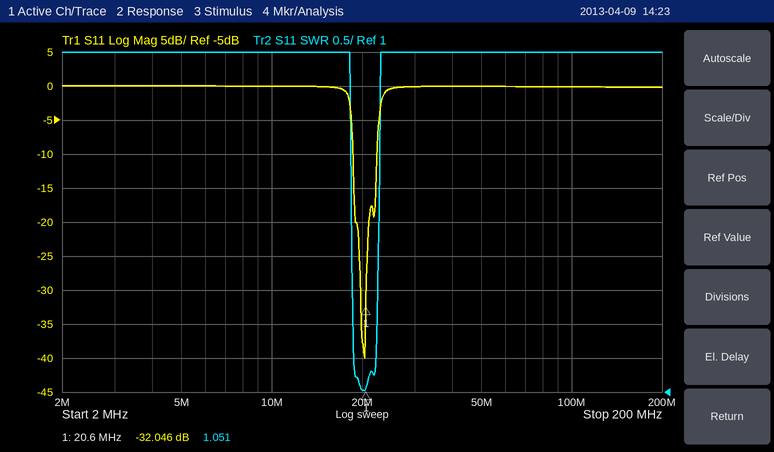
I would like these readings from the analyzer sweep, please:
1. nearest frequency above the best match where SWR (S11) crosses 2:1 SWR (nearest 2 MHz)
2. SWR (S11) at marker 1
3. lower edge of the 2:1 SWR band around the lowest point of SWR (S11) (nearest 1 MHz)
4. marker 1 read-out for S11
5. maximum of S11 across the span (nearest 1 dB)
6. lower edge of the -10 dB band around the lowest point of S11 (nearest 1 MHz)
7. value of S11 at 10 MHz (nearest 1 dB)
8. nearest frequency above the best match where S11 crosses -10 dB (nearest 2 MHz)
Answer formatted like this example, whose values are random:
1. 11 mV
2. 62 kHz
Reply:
1. 22 MHz
2. 1.051
3. 19 MHz
4. -32.046 dB
5. 0 dB
6. 19 MHz
7. 0 dB
8. 22 MHz
